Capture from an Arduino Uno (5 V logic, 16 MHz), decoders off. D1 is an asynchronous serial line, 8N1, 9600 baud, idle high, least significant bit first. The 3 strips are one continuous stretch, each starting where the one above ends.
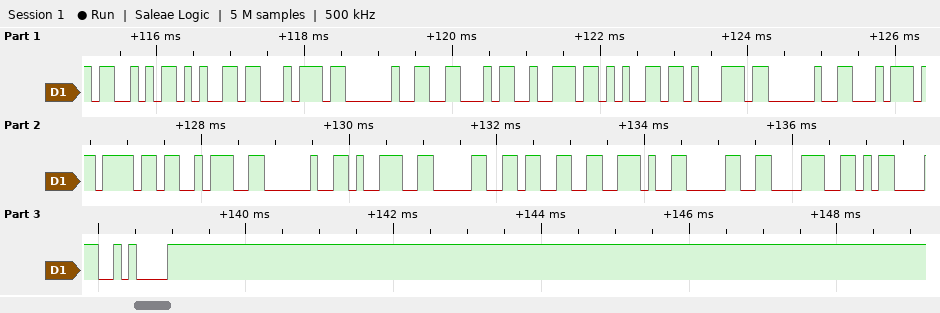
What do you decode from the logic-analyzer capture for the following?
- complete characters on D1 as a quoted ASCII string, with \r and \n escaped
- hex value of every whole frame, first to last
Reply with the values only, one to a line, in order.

"Set Freq to: 903.08\r\n"
53 65 74 20 46 72 65 71 20 74 6F 3A 20 39 30 33 2E 30 38 0D 0A
